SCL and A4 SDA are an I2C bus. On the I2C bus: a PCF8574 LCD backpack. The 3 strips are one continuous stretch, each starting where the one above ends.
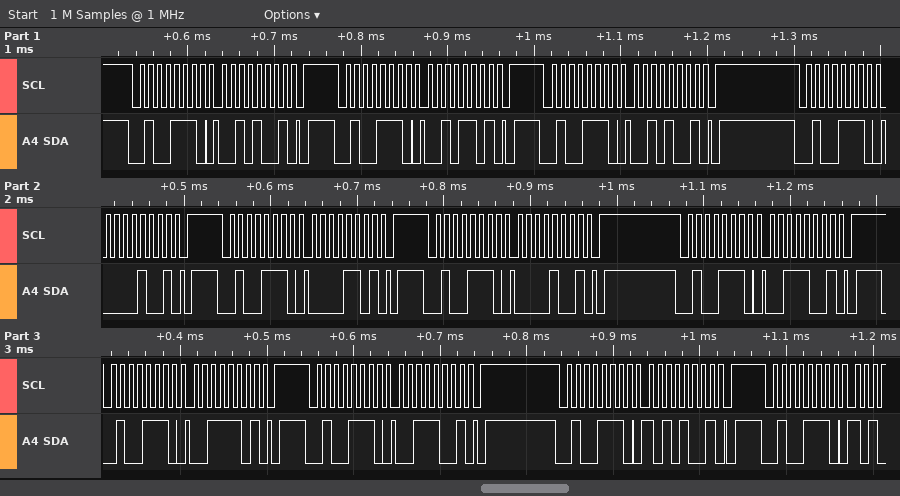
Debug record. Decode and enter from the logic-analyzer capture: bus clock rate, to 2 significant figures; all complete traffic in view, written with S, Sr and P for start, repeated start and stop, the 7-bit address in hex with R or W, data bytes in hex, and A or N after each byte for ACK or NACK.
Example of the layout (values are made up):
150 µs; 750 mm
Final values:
100 kHz; S 27W A 29 A P S 27W A 2D A P S 27W A 29 A P S 27W A 09 A P S 27W A 0D A P S 27W A 09 A P S 27W A 39 A P S 27W A 3D A P S 27W A 39 A P S 27W A A9 A P S 27W A
